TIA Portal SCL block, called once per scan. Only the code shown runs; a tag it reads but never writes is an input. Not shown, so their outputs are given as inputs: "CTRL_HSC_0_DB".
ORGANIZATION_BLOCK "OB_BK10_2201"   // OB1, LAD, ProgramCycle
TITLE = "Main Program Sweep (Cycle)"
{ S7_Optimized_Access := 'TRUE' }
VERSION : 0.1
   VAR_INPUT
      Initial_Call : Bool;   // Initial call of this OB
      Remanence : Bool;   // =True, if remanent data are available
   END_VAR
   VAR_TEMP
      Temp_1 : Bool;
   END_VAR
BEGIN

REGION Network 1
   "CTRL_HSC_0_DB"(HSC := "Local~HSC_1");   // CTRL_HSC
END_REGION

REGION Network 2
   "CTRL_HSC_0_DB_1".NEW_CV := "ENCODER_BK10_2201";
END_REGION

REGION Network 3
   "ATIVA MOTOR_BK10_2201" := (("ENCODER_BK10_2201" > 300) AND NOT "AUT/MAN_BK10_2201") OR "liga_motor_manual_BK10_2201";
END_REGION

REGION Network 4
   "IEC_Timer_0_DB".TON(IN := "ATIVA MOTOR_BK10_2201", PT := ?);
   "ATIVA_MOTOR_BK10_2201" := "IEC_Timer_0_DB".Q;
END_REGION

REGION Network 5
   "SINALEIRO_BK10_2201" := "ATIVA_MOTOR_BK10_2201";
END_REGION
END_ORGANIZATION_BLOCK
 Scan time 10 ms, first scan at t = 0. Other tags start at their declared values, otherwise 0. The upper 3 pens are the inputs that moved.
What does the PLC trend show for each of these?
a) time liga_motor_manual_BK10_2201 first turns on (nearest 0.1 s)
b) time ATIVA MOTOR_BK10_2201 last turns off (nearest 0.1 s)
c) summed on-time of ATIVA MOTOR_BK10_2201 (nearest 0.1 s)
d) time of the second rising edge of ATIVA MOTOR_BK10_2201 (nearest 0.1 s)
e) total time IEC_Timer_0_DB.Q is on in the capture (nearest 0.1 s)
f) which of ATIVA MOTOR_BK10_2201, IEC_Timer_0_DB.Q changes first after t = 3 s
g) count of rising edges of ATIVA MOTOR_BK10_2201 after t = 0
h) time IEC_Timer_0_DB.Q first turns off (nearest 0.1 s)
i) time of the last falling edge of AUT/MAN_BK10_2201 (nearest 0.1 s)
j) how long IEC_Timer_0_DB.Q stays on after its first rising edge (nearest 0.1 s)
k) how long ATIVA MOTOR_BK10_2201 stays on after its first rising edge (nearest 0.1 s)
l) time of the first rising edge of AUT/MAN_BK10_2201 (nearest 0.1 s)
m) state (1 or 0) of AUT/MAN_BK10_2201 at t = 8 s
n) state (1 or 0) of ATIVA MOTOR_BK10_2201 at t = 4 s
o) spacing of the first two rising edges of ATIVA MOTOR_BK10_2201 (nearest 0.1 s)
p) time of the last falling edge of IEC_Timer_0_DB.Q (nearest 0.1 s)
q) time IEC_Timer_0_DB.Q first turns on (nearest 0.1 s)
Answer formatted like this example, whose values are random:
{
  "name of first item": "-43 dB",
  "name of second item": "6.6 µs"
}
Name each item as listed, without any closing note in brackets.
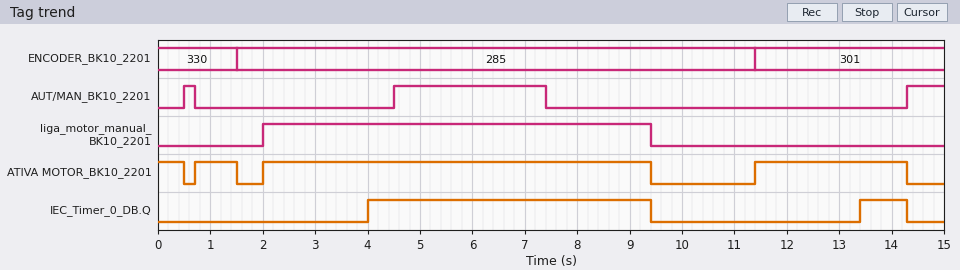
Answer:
{
  "time liga_motor_manual_BK10_2201 first turns on": "2.0 s",
  "time ATIVA MOTOR_BK10_2201 last turns off": "14.3 s",
  "summed on-time of ATIVA MOTOR_BK10_2201": "11.6 s",
  "time of the second rising edge of ATIVA MOTOR_BK10_2201": "2.0 s",
  "total time IEC_Timer_0_DB.Q is on in the capture": "6.3 s",
  "which of ATIVA MOTOR_BK10_2201, IEC_Timer_0_DB.Q changes first after t = 3 s": "IEC_Timer_0_DB.Q",
  "count of rising edges of ATIVA MOTOR_BK10_2201 after t = 0": "3",
  "time IEC_Timer_0_DB.Q first turns off": "9.4 s",
  "time of the last falling edge of AUT/MAN_BK10_2201": "7.4 s",
  "how long IEC_Timer_0_DB.Q stays on after its first rising edge": "5.4 s",
  "how long ATIVA MOTOR_BK10_2201 stays on after its first rising edge": "0.8 s",
  "time of the first rising edge of AUT/MAN_BK10_2201": "0.5 s",
  "state (1 or 0) of AUT/MAN_BK10_2201 at t = 8 s": "0",
  "state (1 or 0) of ATIVA MOTOR_BK10_2201 at t = 4 s": "1",
  "spacing of the first two rising edges of ATIVA MOTOR_BK10_2201": "1.3 s",
  "time of the last falling edge of IEC_Timer_0_DB.Q": "14.3 s",
  "time IEC_Timer_0_DB.Q first turns on": "4.0 s"
}
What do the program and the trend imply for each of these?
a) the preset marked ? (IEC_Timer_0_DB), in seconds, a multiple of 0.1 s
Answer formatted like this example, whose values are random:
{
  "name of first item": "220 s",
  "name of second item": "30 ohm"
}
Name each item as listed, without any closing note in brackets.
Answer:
{
  "the preset marked ? (IEC_Timer_0_DB), in seconds, a multiple of 0.1 s": "2.0 s"
}
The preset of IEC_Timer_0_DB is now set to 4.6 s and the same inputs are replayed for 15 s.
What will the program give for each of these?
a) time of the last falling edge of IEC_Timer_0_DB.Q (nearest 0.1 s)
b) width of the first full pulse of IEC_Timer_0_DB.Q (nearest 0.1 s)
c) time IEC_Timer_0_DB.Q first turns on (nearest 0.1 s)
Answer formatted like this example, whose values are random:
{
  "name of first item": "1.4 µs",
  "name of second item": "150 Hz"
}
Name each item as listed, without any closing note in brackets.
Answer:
{
  "time of the last falling edge of IEC_Timer_0_DB.Q": "9.4 s",
  "width of the first full pulse of IEC_Timer_0_DB.Q": "2.8 s",
  "time IEC_Timer_0_DB.Q first turns on": "6.6 s"
}
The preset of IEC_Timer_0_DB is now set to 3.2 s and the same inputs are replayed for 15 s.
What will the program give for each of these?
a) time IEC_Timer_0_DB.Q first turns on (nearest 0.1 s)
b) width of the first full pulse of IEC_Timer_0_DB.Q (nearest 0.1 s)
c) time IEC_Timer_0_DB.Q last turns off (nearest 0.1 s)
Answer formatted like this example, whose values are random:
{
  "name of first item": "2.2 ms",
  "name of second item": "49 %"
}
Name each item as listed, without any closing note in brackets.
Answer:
{
  "time IEC_Timer_0_DB.Q first turns on": "5.2 s",
  "width of the first full pulse of IEC_Timer_0_DB.Q": "4.2 s",
  "time IEC_Timer_0_DB.Q last turns off": "9.4 s"
}
